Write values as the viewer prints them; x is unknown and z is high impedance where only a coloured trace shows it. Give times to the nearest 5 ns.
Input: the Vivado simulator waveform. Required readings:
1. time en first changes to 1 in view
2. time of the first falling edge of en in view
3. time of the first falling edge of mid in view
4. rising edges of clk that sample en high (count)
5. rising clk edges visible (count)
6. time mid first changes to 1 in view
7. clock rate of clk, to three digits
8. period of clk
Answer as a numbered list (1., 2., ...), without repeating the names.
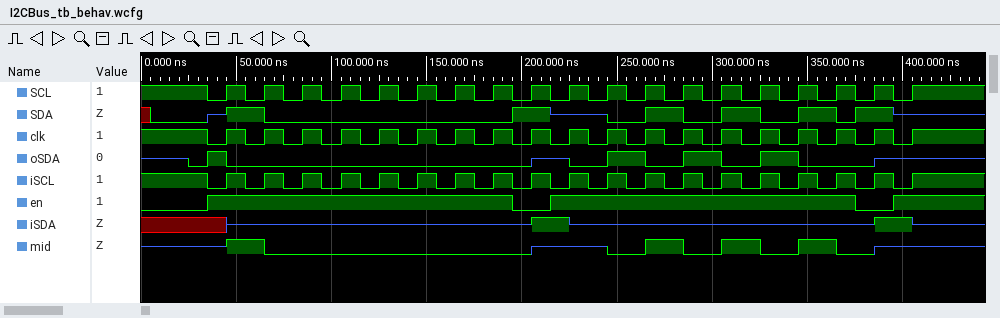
1. 35 ns
2. 195 ns
3. 65 ns
4. 17
5. 19
6. 45 ns
7. 50.0 MHz
8. 20 ns
